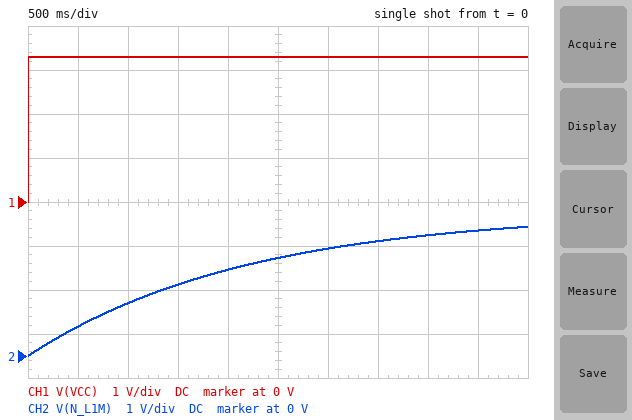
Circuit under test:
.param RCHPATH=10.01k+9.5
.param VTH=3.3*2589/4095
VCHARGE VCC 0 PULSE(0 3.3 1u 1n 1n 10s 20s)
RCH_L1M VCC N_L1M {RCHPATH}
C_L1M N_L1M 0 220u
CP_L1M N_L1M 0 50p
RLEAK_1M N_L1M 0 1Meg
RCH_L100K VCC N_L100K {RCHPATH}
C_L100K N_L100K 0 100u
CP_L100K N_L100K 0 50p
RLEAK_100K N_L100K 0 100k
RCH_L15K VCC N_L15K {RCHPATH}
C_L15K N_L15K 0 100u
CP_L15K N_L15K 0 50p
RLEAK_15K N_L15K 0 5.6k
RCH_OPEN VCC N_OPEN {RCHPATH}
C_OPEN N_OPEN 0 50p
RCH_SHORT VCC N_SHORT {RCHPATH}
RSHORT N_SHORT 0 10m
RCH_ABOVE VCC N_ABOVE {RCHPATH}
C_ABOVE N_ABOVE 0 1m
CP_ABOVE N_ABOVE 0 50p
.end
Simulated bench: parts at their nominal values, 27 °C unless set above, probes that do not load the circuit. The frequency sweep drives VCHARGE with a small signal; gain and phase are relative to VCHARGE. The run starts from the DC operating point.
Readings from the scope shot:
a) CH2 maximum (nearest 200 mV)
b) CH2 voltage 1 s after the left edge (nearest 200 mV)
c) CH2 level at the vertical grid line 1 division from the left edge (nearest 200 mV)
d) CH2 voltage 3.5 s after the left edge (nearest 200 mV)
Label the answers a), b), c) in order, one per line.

a) 3.0 V
b) 1.2 V
c) 600 mV
d) 2.6 V
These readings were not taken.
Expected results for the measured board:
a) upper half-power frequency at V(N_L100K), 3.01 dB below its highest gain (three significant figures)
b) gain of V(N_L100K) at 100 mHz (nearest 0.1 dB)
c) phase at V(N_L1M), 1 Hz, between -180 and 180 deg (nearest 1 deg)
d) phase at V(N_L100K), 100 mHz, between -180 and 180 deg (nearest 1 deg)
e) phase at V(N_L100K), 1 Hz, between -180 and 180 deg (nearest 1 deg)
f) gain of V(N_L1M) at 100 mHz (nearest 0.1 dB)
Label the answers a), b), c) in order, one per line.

a) 175 mHz
b) -2.1 dB
c) -86 deg
d) -30 deg
e) -80 deg
f) -4.7 dB
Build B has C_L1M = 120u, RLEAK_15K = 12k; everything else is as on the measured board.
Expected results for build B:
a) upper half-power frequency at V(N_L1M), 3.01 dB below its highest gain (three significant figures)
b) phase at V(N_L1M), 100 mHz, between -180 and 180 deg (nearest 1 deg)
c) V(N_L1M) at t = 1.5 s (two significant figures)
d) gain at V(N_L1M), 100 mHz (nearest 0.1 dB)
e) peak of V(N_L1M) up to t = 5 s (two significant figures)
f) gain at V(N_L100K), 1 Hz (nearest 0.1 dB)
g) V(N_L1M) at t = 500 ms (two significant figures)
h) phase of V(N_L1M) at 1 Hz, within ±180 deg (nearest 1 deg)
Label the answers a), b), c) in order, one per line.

a) 134 mHz
b) -37 deg
c) 2.3 V
d) -2.0 dB
e) 3.2 V
f) -16.1 dB
g) 1.1 V
h) -82 deg
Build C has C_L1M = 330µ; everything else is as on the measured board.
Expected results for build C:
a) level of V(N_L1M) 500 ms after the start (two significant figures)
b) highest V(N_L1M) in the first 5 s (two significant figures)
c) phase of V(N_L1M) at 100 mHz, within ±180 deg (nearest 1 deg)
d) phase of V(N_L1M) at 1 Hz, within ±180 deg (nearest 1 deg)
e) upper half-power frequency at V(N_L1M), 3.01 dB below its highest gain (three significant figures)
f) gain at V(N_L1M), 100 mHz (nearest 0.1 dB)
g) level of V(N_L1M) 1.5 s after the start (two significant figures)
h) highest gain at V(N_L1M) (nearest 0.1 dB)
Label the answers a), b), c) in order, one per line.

a) 460 mV
b) 2.6 V
c) -64 deg
d) -87 deg
e) 48.6 mHz
f) -7.3 dB
g) 1.2 V
h) -0.1 dB
